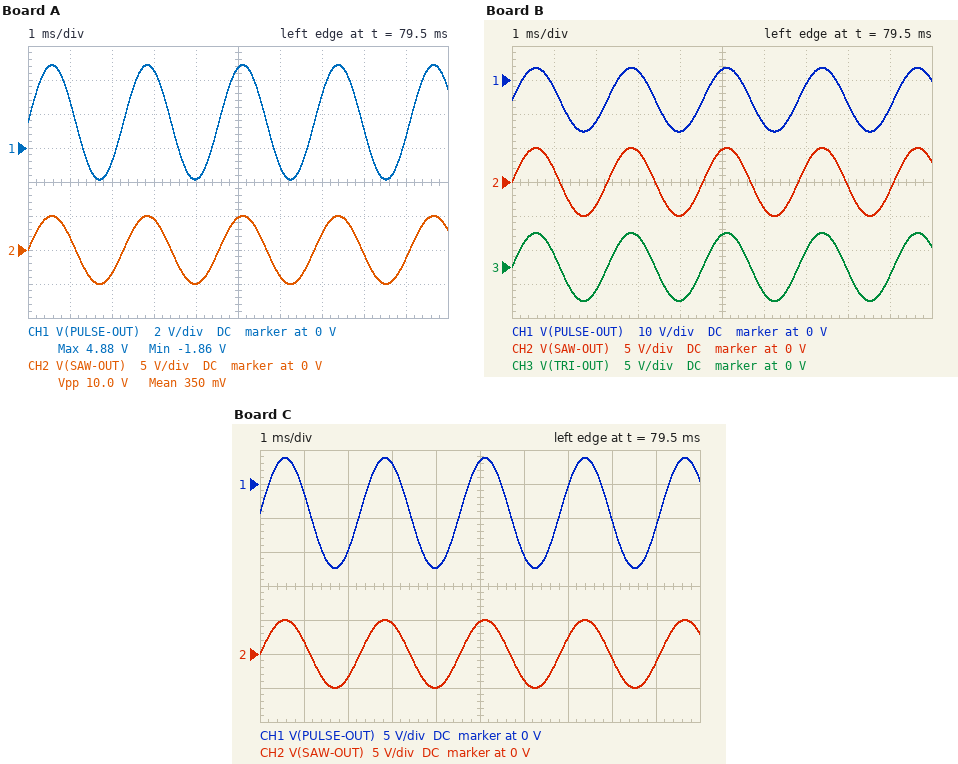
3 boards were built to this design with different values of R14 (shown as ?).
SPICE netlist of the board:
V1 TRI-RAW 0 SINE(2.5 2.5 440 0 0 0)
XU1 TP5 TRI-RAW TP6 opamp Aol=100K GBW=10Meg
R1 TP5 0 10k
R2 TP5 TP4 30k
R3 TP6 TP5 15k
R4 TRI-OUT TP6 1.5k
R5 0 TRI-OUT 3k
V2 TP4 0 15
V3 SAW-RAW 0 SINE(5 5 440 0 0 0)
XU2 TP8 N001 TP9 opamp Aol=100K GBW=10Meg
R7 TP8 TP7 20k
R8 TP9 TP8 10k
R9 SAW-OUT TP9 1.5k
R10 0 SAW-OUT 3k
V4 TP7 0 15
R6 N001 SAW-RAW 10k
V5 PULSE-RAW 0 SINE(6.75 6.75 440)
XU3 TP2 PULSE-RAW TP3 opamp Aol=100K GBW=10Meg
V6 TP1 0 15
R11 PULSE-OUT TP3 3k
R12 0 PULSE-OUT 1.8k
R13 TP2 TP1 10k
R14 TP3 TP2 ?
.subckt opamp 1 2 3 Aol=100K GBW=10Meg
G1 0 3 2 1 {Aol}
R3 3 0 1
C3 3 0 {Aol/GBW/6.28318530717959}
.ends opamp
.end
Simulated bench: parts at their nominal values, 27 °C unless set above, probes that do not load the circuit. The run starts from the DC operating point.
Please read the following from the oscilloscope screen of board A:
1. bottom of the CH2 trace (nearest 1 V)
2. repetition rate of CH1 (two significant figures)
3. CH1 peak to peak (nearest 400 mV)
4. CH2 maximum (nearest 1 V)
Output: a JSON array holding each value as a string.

["-5 V", "440 Hz", "6.8 V", "5 V"]
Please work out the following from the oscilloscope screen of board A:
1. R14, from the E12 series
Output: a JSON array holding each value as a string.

["3.3 kΩ"]
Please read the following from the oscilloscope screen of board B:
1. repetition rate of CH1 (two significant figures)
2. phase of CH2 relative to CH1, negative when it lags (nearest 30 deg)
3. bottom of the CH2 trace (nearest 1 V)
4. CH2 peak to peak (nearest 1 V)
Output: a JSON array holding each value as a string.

["440 Hz", "0 deg", "-5 V", "10 V"]
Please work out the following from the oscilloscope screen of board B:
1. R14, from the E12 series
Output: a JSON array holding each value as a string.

["27 kΩ"]
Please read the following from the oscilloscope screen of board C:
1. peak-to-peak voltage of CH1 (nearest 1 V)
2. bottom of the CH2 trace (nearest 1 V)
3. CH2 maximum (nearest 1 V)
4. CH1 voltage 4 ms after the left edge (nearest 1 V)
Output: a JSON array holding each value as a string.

["16 V", "-5 V", "5 V", "-12 V"]
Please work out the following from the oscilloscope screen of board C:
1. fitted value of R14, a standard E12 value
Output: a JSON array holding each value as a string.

["22 kΩ"]
